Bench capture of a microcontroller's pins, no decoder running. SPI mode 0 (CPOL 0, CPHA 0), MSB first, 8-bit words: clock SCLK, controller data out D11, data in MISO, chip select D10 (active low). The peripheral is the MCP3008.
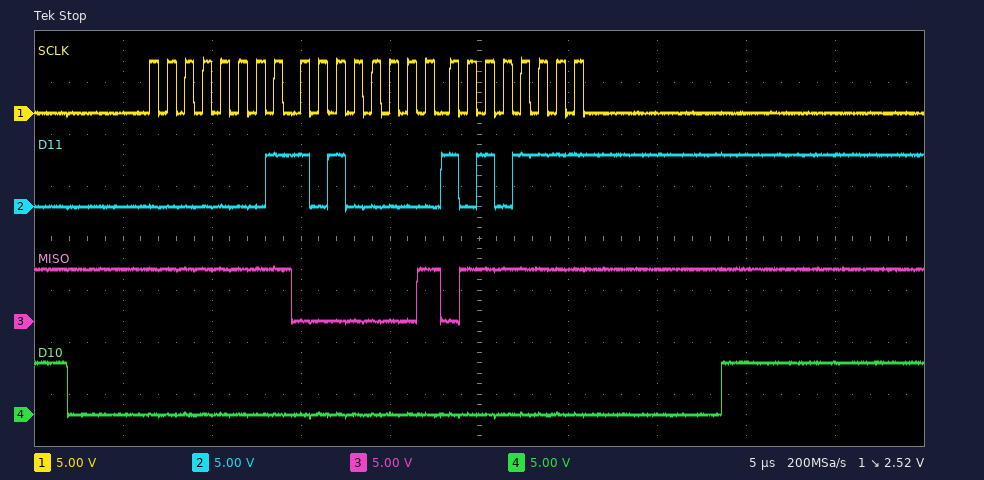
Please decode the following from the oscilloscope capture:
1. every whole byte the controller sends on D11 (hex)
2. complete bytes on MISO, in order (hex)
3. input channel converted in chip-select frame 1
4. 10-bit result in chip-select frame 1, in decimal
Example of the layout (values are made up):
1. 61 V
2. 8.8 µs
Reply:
1. 01 A0 AF
2. FF 01 7F
3. 2
4. 383
